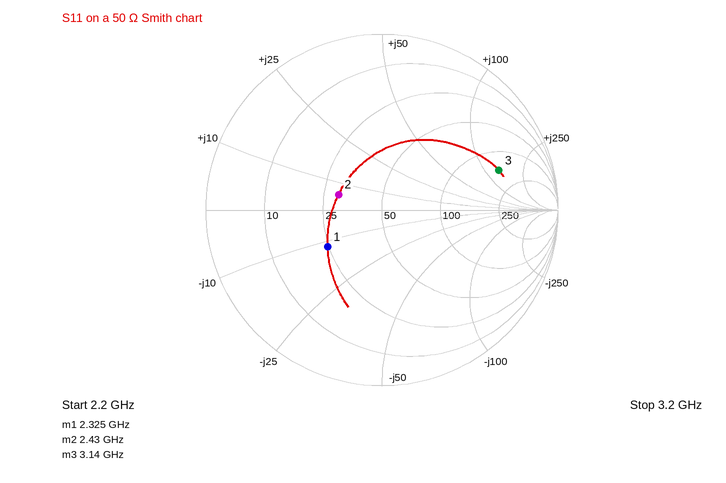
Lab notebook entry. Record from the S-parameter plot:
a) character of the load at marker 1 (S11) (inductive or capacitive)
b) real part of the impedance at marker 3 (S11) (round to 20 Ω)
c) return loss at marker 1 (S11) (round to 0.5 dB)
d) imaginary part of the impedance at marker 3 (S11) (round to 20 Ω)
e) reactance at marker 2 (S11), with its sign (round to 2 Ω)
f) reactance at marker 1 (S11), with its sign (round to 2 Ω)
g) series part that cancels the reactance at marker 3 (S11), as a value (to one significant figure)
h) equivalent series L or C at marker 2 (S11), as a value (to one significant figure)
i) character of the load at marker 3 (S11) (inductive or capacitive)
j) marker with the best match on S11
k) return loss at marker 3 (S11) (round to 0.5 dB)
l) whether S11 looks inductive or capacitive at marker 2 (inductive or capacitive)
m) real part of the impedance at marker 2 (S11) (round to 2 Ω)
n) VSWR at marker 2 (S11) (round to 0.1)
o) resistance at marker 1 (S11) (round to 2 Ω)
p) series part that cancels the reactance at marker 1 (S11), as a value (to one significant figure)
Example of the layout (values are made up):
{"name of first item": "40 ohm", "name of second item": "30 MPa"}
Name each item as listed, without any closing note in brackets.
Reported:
{"character of the load at marker 1 (S11)": "capacitive", "real part of the impedance at marker 3 (S11)": "160 Ω", "return loss at marker 1 (S11)": "8.5 dB", "imaginary part of the impedance at marker 3 (S11)": "+140 Ω", "reactance at marker 2 (S11), with its sign": "+6 Ω", "reactance at marker 1 (S11), with its sign": "-12 Ω", "series part that cancels the reactance at marker 3 (S11), as a value": "400 fF", "equivalent series L or C at marker 2 (S11), as a value": "400 pH", "character of the load at marker 3 (S11)": "inductive", "marker with the best match on S11": "marker 2", "return loss at marker 3 (S11)": "3.0 dB", "whether S11 looks inductive or capacitive at marker 2": "inductive", "real part of the impedance at marker 2 (S11)": "30 Ω", "VSWR at marker 2 (S11)": "1.7", "resistance at marker 1 (S11)": "24 Ω", "series part that cancels the reactance at marker 1 (S11), as a value": "800 pH"}
